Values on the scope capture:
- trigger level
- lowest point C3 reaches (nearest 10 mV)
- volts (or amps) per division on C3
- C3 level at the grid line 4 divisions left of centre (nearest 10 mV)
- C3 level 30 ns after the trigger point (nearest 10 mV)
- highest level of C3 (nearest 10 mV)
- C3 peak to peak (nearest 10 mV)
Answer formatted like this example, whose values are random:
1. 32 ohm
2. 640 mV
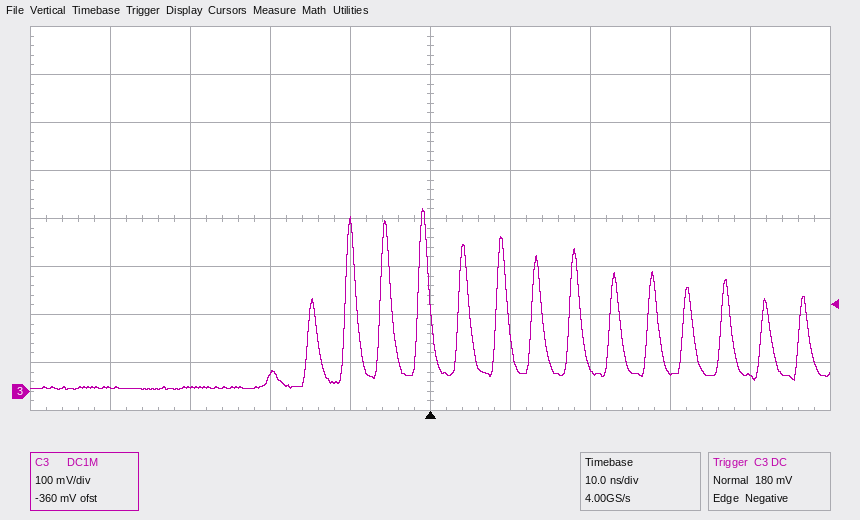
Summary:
1. 180 mV
2. 0 mV
3. 100 mV
4. 10 mV
5. 40 mV
6. 380 mV
7. 380 mV
